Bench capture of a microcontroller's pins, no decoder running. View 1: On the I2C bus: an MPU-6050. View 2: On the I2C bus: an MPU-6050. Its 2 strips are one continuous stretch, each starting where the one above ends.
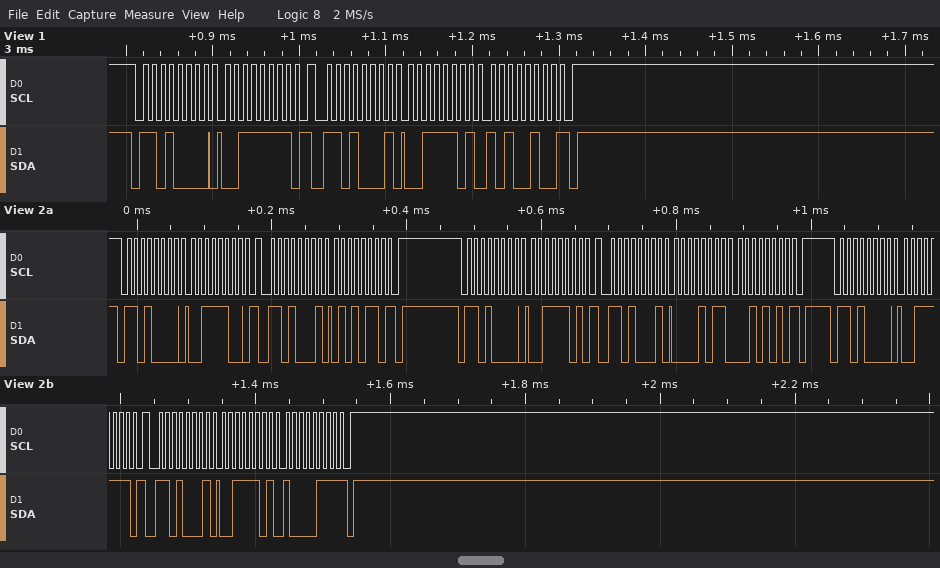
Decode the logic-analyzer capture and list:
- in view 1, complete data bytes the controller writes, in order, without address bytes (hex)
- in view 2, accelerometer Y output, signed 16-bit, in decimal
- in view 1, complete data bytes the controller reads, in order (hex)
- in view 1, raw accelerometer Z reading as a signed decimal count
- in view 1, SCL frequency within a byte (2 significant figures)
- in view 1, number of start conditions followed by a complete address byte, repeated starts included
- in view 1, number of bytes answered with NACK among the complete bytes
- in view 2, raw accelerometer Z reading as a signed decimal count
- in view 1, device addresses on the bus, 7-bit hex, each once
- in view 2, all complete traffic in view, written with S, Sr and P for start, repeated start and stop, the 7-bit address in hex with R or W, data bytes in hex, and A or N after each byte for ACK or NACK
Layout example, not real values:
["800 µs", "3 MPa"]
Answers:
["3F", "2858", "3D A4", "15780", "100 kHz", "2", "1", "15751", "0x68", "S 68W A 3C A Sr 68R A 56 N P S 68W A 3D A Sr 68R A 0B A 2A N P S 68W A 3F A Sr 68R A 3D A 87 N P"]
